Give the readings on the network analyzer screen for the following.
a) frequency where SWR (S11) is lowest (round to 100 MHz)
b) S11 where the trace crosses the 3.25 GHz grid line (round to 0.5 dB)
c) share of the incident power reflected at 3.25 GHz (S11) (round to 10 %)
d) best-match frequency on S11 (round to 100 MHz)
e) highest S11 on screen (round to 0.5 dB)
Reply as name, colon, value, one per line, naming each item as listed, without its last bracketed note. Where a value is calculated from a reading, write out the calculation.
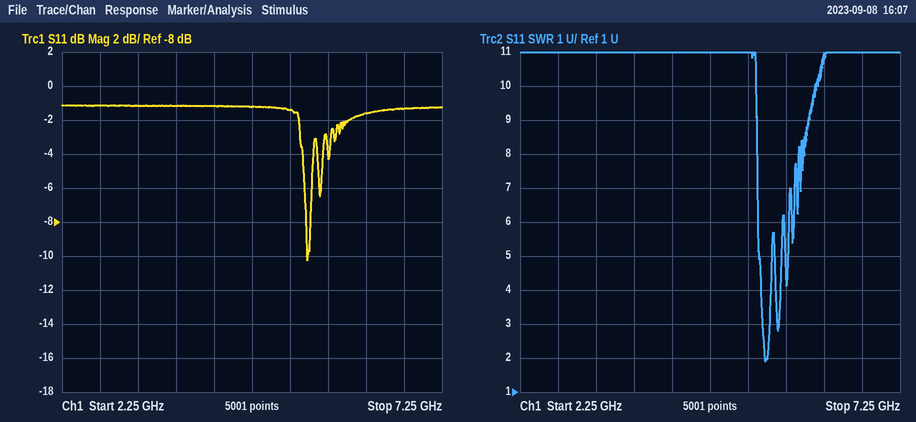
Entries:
frequency where SWR (S11) is lowest: 5.5 GHz
S11 where the trace crosses the 3.25 GHz grid line: -1.0 dB
share of the incident power reflected at 3.25 GHz (S11): 10^(-1/10) ≈ 79.4 %, so 80 % to the nearest 10 %
best-match frequency on S11: 5.5 GHz
highest S11 on screen: -1.0 dB
